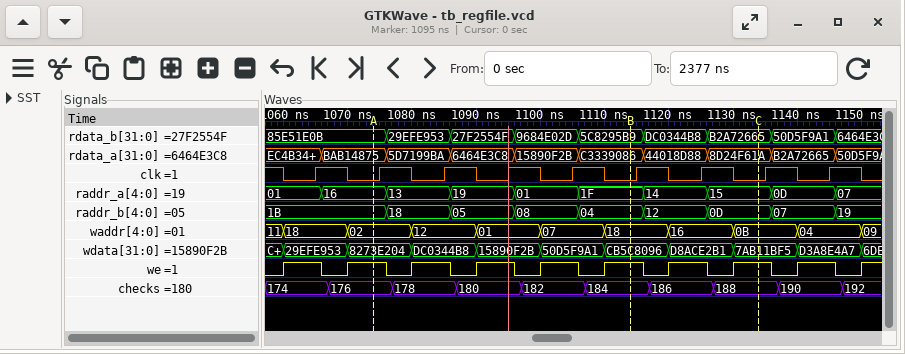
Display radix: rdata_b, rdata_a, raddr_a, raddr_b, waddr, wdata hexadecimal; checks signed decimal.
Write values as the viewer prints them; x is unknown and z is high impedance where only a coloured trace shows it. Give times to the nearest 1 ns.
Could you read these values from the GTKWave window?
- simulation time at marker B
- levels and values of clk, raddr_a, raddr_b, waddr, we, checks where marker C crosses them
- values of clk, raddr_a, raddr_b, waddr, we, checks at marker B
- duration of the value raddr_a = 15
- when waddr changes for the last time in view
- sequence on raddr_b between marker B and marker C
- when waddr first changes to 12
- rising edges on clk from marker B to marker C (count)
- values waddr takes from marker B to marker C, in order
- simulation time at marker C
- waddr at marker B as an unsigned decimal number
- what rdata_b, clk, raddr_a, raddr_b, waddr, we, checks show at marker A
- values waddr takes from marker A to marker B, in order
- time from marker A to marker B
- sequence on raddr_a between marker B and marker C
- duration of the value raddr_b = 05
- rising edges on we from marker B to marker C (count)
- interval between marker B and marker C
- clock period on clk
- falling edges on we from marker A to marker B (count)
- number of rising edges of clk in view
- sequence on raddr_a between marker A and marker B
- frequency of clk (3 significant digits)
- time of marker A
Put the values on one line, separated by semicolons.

1114 ns; clk=0, raddr_a=15, raddr_b=0D, waddr=0B, we=1, checks=188; clk=0, raddr_a=1F, raddr_b=04, waddr=18, we=1, checks=184; 10 ns; 1150 ns; 04, 12, 0D; 1080 ns; 2; 18, 16, 0B; 1134 ns; 24; rdata_b=85E51E0B, clk=0, raddr_a=16, raddr_b=1B, waddr=02, we=1, checks=176; 02, 12, 01, 07, 18; 40 ns; 1F, 14, 15; 10 ns; 2; 20 ns; 10 ns; 4; 9; 16, 13, 19, 01, 1F; 100 MHz; 1074 ns
